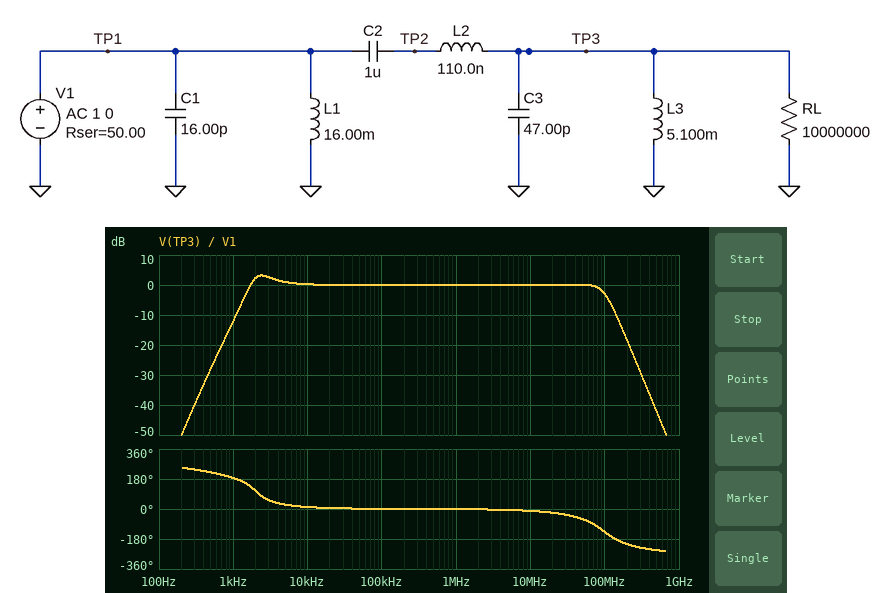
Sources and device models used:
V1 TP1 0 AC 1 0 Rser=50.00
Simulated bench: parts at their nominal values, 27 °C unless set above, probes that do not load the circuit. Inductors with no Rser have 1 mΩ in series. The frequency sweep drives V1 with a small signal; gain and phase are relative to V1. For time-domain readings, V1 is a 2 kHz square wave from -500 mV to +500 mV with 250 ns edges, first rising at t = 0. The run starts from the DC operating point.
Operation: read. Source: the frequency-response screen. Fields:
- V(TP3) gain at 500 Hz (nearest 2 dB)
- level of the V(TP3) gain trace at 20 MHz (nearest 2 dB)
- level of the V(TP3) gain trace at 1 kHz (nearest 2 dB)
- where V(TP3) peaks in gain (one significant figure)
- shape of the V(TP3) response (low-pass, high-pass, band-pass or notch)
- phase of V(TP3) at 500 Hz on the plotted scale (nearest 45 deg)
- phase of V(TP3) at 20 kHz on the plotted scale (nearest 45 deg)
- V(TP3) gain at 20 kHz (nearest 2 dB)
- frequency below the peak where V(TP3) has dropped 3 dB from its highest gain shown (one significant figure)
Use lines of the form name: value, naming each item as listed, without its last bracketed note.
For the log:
V(TP3) gain at 500 Hz: -28 dB
level of the V(TP3) gain trace at 20 MHz: 0 dB
level of the V(TP3) gain trace at 1 kHz: -12 dB
where V(TP3) peaks in gain: 2 kHz
shape of the V(TP3) response: band-pass
phase of V(TP3) at 500 Hz on the plotted scale: 225 deg
phase of V(TP3) at 20 kHz on the plotted scale: 0 deg
V(TP3) gain at 20 kHz: 0 dB
frequency below the peak where V(TP3) has dropped 3 dB from its highest gain shown: 2 kHz
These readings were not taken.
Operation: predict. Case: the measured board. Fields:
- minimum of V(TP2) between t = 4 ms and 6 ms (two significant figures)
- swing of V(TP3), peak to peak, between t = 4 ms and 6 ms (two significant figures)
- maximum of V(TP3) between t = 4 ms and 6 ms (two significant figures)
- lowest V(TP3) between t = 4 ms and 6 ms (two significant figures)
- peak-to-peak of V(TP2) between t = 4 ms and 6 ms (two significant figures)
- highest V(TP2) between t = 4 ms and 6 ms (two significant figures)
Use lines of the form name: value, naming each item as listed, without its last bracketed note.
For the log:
minimum of V(TP2) between t = 4 ms and 6 ms: -1.5 V
swing of V(TP3), peak to peak, between t = 4 ms and 6 ms: 2.9 V
maximum of V(TP3) between t = 4 ms and 6 ms: 1.5 V
lowest V(TP3) between t = 4 ms and 6 ms: -1.5 V
peak-to-peak of V(TP2) between t = 4 ms and 6 ms: 2.9 V
highest V(TP2) between t = 4 ms and 6 ms: 1.5 V
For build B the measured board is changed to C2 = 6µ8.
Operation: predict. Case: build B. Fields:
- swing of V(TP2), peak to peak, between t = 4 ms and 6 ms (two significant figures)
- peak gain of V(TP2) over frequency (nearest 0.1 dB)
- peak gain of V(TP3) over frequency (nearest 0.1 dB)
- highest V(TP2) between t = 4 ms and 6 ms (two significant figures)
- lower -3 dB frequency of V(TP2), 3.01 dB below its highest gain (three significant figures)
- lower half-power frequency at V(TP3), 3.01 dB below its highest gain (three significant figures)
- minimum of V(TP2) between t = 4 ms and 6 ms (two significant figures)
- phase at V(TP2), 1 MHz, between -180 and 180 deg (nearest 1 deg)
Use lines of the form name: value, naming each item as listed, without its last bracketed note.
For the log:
swing of V(TP2), peak to peak, between t = 4 ms and 6 ms: 2.1 V
peak gain of V(TP2) over frequency: 0 dB
peak gain of V(TP3) over frequency: 0.1 dB
highest V(TP2) between t = 4 ms and 6 ms: 1.0 V
lower -3 dB frequency of V(TP2), 3.01 dB below its highest gain: 1.55 kHz
lower half-power frequency at V(TP3), 3.01 dB below its highest gain: 1.59 kHz
minimum of V(TP2) between t = 4 ms and 6 ms: -1.0 V
phase at V(TP2), 1 MHz, between -180 and 180 deg: -1 deg
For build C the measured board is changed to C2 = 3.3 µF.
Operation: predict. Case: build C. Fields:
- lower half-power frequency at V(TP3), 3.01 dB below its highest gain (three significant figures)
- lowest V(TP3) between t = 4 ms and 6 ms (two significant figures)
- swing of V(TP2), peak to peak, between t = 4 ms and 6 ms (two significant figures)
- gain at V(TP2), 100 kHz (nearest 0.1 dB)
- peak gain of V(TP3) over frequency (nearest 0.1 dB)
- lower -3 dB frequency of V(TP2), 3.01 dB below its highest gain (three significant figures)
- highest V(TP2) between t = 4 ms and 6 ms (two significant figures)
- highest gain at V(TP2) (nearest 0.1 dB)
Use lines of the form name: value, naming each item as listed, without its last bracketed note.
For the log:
lower half-power frequency at V(TP3), 3.01 dB below its highest gain: 1.00 kHz
lowest V(TP3) between t = 4 ms and 6 ms: -1.1 V
swing of V(TP2), peak to peak, between t = 4 ms and 6 ms: 2.2 V
gain at V(TP2), 100 kHz: 0 dB
peak gain of V(TP3) over frequency: 0.1 dB
lower -3 dB frequency of V(TP2), 3.01 dB below its highest gain: 988 Hz
highest V(TP2) between t = 4 ms and 6 ms: 1.1 V
highest gain at V(TP2): 0 dB
